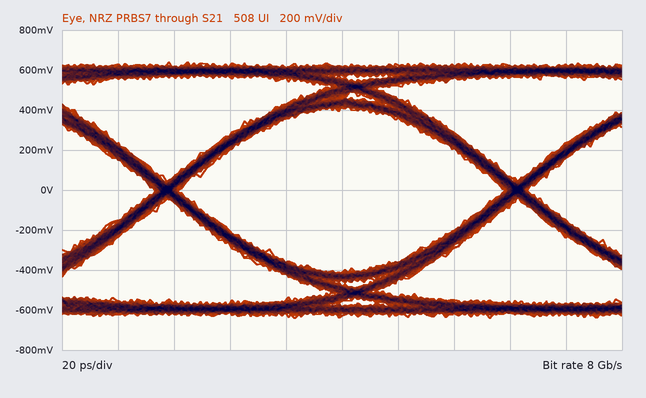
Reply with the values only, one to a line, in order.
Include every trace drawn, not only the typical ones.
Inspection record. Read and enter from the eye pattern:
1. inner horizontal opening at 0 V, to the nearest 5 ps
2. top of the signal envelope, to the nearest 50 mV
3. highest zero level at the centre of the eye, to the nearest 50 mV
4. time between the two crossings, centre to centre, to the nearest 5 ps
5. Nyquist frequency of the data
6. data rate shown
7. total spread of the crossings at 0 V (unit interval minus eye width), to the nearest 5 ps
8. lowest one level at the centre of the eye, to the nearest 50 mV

115 ps
650 mV
-400 mV
125 ps
4 GHz
8 Gb/s
10 ps
400 mV
